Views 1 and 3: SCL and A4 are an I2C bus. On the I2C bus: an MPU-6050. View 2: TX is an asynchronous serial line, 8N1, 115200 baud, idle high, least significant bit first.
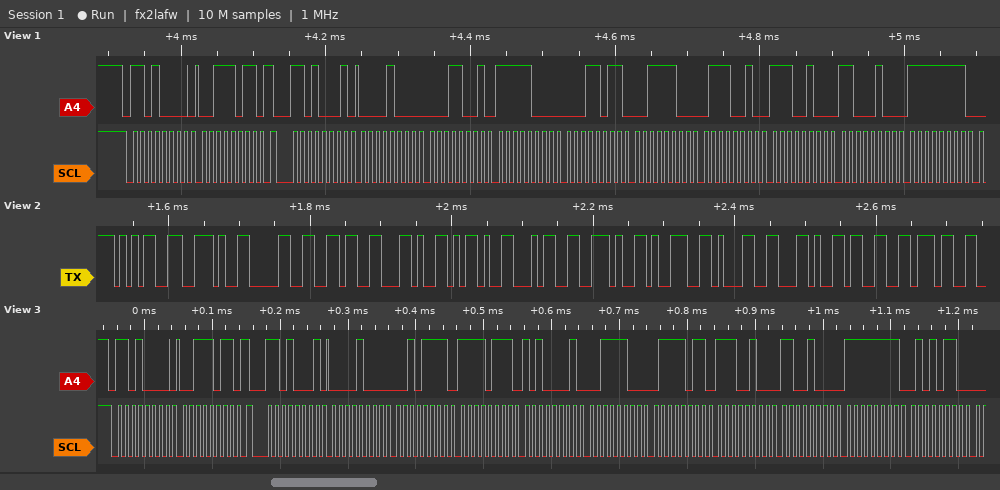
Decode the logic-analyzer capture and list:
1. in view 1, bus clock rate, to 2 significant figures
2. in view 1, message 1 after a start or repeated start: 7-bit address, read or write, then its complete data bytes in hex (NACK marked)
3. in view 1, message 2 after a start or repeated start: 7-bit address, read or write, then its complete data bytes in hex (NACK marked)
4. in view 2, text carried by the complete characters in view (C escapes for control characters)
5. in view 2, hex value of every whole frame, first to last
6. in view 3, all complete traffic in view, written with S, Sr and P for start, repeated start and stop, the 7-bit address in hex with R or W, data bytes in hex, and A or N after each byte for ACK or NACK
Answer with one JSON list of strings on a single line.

["100 kHz", "0x68 write: 3B", "0x68 read: 08 19 F8 1B 3C 72 E4 C4 FF", "\"5.06,-4.91,37\"", "35 2E 30 36 2C 2D 34 2E 39 31 2C 33 37", "S 68W A 3B A Sr 68R A 08 A 2F A F7 A A1 A 3C A 7B A E4 A C8 A FF A 56 A"]
